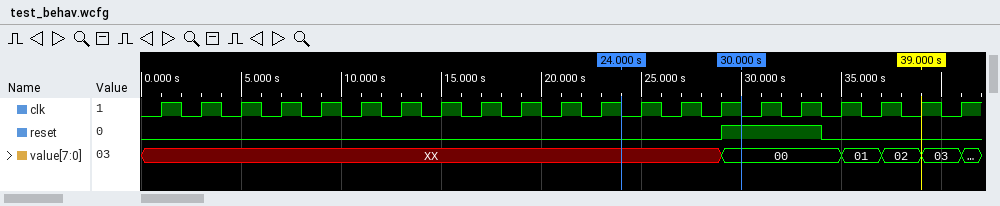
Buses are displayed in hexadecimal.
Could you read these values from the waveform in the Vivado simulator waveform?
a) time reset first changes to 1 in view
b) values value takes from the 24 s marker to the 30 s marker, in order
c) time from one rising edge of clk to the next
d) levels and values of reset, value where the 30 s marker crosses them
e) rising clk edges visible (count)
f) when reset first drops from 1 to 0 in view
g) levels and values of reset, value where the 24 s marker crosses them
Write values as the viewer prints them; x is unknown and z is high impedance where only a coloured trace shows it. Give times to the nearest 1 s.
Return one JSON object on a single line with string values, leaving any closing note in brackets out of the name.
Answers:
{"time reset first changes to 1 in view": "29 s", "values value takes from the 24 s marker to the 30 s marker, in order": "XX, 00", "time from one rising edge of clk to the next": "2 s", "levels and values of reset, value where the 30 s marker crosses them": "reset=1, value=00", "rising clk edges visible": "21", "when reset first drops from 1 to 0 in view": "34 s", "levels and values of reset, value where the 24 s marker crosses them": "reset=0, value=XX"}
